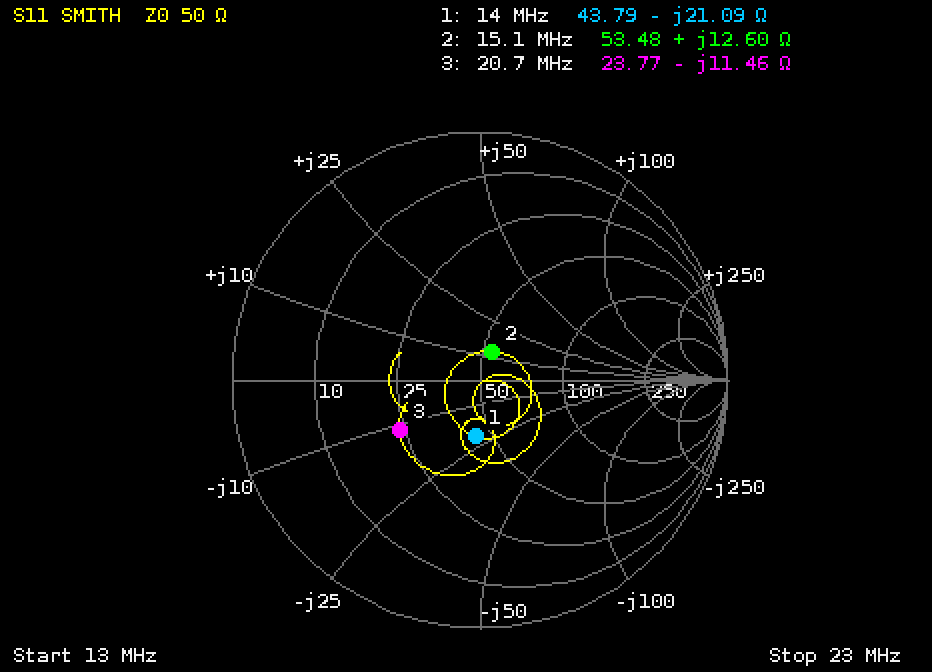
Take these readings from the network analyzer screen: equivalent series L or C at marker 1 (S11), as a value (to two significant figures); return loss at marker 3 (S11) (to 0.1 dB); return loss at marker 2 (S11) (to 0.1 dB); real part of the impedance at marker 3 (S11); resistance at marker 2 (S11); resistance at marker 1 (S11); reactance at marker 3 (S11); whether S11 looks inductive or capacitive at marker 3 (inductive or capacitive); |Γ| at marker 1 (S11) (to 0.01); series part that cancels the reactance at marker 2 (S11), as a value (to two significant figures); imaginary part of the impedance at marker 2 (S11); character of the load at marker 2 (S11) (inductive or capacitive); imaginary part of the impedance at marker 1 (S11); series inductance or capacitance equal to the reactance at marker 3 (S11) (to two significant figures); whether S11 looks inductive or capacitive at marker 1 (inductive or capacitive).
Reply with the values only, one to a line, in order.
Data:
540 pF
8.3 dB
18.0 dB
23.77 Ω
53.48 Ω
43.79 Ω
-11.46 Ω
capacitive
0.23
840 pF
+12.60 Ω
inductive
-21.09 Ω
670 pF
capacitive
